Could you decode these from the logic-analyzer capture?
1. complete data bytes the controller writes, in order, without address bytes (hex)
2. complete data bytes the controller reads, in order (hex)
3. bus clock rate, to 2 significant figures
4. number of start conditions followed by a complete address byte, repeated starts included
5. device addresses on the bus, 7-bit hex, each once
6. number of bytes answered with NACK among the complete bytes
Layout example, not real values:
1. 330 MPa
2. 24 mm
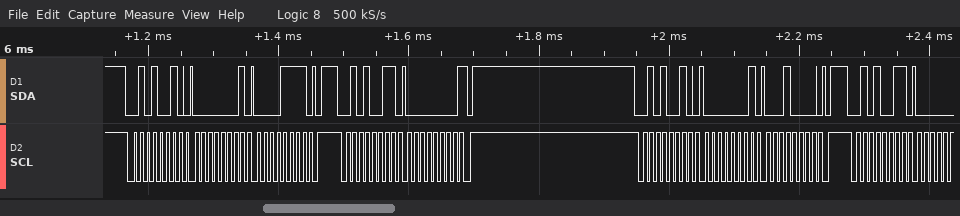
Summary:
1. 01 0F 01 10
2. 00
3. 100 kHz
4. 4
5. 0x29
6. 1
